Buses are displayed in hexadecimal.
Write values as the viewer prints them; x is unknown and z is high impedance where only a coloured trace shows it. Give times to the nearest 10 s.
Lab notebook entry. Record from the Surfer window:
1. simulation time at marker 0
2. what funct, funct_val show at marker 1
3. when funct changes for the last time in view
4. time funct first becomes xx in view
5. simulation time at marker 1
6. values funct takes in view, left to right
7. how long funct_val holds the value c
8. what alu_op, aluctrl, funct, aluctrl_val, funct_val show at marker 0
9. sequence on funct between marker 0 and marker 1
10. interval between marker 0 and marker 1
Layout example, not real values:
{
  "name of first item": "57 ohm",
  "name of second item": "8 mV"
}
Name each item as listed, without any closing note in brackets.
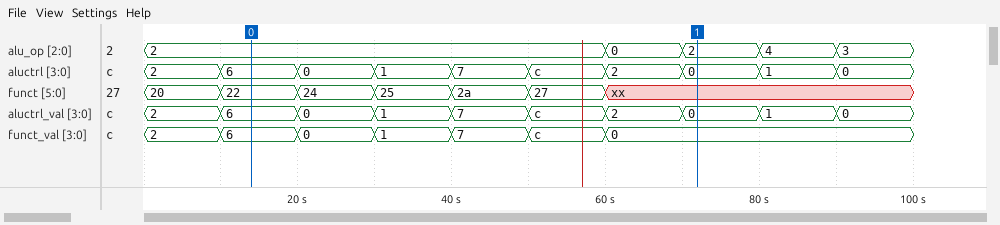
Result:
{
  "simulation time at marker 0": "10 s",
  "what funct, funct_val show at marker 1": "funct=xx, funct_val=0",
  "when funct changes for the last time in view": "60 s",
  "time funct first becomes xx in view": "60 s",
  "simulation time at marker 1": "70 s",
  "values funct takes in view, left to right": "20, 22, 24, 25, 2a, 27, xx",
  "how long funct_val holds the value c": "10 s",
  "what alu_op, aluctrl, funct, aluctrl_val, funct_val show at marker 0": "alu_op=2, aluctrl=6, funct=22, aluctrl_val=6, funct_val=6",
  "sequence on funct between marker 0 and marker 1": "22, 24, 25, 2a, 27, xx",
  "interval between marker 0 and marker 1": "60 s"
}
